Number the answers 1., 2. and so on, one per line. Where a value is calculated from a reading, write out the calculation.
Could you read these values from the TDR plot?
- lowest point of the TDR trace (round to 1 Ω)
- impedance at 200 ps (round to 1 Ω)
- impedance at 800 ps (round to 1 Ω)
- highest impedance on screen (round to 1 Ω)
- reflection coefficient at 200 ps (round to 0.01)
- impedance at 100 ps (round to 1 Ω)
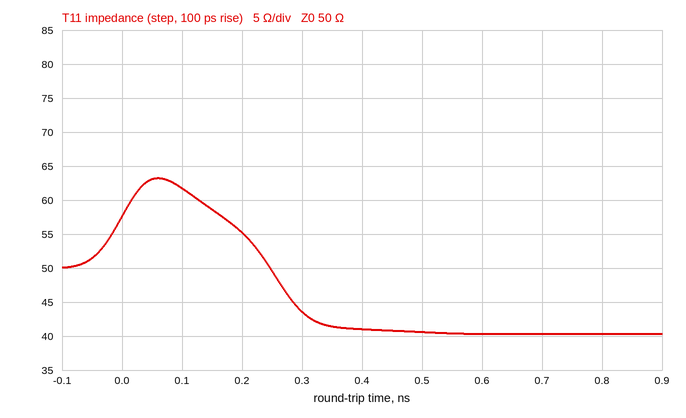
1. 40 Ω
2. 55 Ω
3. 40 Ω
4. 63 Ω
5. (55 − 50)/(55 + 50) ≈ +0.05
6. 62 Ω
